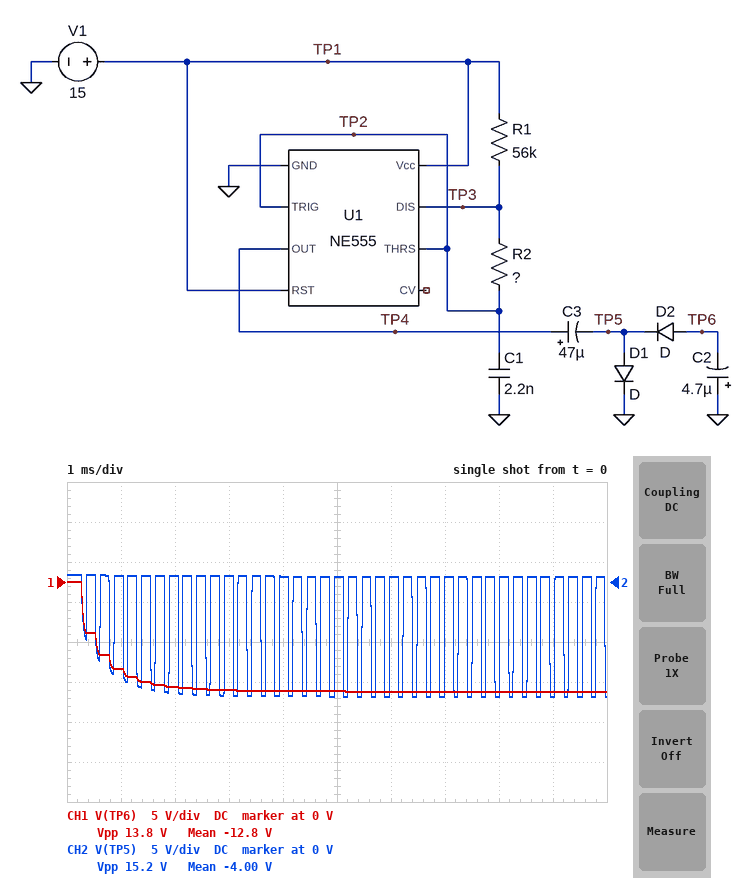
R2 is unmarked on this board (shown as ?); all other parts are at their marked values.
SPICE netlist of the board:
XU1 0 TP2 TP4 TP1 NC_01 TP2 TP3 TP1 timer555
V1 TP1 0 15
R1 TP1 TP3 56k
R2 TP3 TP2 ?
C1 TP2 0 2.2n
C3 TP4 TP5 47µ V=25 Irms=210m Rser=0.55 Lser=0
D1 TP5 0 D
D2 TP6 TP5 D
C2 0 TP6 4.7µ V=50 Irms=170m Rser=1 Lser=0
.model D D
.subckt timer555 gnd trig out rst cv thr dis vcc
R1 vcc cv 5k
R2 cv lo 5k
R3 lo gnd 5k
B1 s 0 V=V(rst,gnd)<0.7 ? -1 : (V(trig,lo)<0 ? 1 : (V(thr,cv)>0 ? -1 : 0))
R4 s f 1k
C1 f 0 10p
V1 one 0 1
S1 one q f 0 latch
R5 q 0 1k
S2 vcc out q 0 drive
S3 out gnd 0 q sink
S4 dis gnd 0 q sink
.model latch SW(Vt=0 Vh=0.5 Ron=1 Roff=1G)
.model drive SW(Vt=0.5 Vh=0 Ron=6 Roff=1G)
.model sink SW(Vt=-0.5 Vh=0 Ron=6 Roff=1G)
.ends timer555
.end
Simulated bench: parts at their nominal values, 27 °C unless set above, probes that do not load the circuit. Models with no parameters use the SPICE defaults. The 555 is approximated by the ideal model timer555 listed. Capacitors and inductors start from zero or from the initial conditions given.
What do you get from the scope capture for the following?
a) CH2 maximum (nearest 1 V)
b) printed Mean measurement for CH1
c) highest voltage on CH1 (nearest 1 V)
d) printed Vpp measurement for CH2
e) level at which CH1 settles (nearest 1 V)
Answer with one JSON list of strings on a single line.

["1 V", "-12.8 V", "0 V", "15.2 V", "-14 V"]
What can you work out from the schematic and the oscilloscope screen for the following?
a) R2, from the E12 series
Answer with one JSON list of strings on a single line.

["56 kΩ"]
